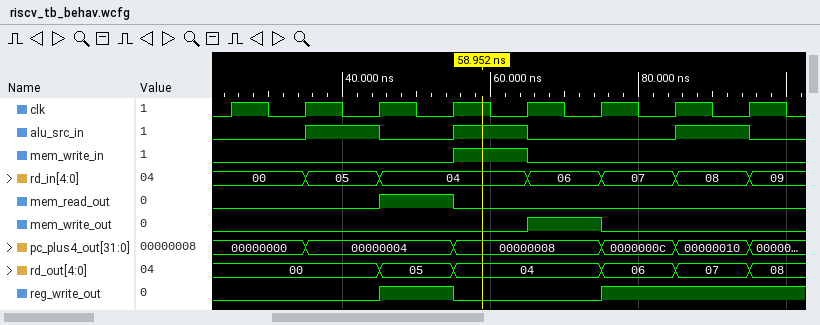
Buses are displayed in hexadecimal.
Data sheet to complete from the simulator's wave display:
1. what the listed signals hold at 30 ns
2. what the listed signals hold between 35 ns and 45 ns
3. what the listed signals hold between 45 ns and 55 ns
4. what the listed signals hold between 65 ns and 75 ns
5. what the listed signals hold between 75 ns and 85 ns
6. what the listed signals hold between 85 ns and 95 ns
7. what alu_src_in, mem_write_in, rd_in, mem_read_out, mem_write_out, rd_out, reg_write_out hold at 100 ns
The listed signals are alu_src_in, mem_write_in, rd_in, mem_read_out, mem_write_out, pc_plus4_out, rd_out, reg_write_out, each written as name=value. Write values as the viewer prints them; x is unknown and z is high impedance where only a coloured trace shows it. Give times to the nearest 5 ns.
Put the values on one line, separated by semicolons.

alu_src_in=0, mem_write_in=0, rd_in=00, mem_read_out=0, mem_write_out=0, pc_plus4_out=00000000, rd_out=00, reg_write_out=0; alu_src_in=1, mem_write_in=0, rd_in=05, mem_read_out=0, mem_write_out=0, pc_plus4_out=00000004, rd_out=00, reg_write_out=0; alu_src_in=0, mem_write_in=0, rd_in=04, mem_read_out=1, mem_write_out=0, pc_plus4_out=00000004, rd_out=05, reg_write_out=1; alu_src_in=0, mem_write_in=0, rd_in=06, mem_read_out=0, mem_write_out=1, pc_plus4_out=00000008, rd_out=04, reg_write_out=0; alu_src_in=0, mem_write_in=0, rd_in=07, mem_read_out=0, mem_write_out=0, pc_plus4_out=0000000c, rd_out=06, reg_write_out=1; alu_src_in=1, mem_write_in=0, rd_in=08, mem_read_out=0, mem_write_out=0, pc_plus4_out=00000010, rd_out=07, reg_write_out=1; alu_src_in=0, mem_write_in=0, rd_in=09, mem_read_out=0, mem_write_out=0, rd_out=08, reg_write_out=1
